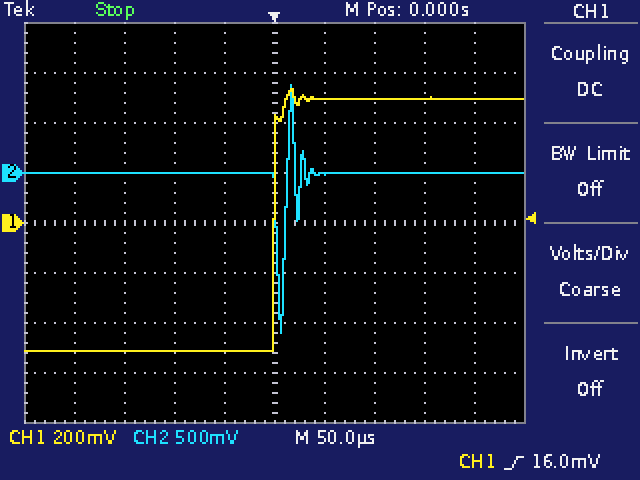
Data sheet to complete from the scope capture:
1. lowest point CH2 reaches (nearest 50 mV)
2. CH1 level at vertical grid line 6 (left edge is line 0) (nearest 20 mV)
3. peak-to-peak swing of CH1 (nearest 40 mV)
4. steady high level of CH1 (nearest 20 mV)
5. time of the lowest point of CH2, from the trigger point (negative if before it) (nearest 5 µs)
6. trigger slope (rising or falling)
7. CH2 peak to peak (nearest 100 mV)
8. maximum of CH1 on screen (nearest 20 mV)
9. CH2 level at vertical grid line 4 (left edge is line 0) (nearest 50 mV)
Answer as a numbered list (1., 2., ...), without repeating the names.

1. -1.60 V
2. 500 mV
3. 1.04 V
4. 500 mV
5. +5 µs
6. rising
7. 2.50 V
8. 540 mV
9. 0 mV
